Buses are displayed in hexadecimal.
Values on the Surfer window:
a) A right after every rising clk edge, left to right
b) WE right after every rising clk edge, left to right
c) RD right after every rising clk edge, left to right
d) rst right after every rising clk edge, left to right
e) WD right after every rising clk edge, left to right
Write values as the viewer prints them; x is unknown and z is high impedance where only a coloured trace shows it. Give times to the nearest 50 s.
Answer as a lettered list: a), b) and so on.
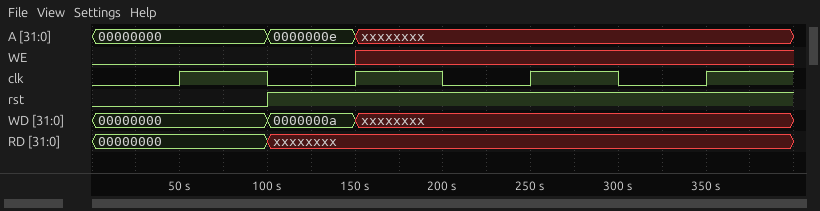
a) 00000000, xxxxxxxx, xxxxxxxx, xxxxxxxx
b) 0 x x x
c) 00000000, xxxxxxxx, xxxxxxxx, xxxxxxxx
d) 0 1 1 1
e) 00000000, xxxxxxxx, xxxxxxxx, xxxxxxxx
